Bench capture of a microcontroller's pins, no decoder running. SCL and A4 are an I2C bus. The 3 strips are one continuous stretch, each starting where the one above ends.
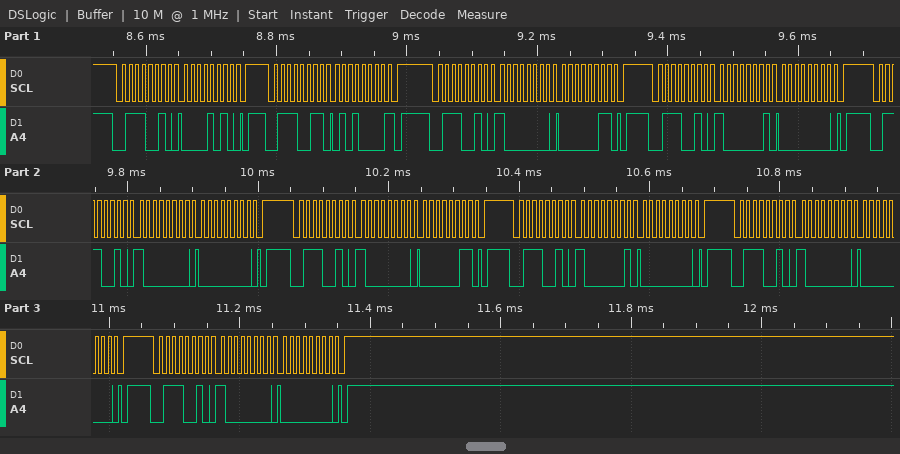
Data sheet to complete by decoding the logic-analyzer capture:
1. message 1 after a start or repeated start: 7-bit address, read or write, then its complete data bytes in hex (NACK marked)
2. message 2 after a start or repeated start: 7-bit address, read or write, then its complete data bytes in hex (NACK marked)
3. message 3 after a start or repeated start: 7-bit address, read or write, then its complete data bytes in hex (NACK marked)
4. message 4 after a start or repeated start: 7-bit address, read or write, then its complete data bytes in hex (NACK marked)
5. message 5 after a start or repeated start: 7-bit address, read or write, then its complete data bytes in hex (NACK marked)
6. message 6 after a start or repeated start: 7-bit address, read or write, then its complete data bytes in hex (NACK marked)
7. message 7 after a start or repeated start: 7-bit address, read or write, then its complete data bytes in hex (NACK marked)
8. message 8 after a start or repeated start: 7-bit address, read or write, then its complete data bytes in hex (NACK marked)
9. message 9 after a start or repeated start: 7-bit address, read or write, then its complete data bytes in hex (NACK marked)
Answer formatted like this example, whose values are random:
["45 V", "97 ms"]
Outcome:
["0x39 write: 0A", "0x39 read: 50 NACK", "0x39 write: 80 03", "0x39 write: 81 00", "0x39 write: 80 00", "0x39 write: 80 03", "0x39 write: 81 00", "0x39 write: 80 00", "0x39 write: 80 00"]
